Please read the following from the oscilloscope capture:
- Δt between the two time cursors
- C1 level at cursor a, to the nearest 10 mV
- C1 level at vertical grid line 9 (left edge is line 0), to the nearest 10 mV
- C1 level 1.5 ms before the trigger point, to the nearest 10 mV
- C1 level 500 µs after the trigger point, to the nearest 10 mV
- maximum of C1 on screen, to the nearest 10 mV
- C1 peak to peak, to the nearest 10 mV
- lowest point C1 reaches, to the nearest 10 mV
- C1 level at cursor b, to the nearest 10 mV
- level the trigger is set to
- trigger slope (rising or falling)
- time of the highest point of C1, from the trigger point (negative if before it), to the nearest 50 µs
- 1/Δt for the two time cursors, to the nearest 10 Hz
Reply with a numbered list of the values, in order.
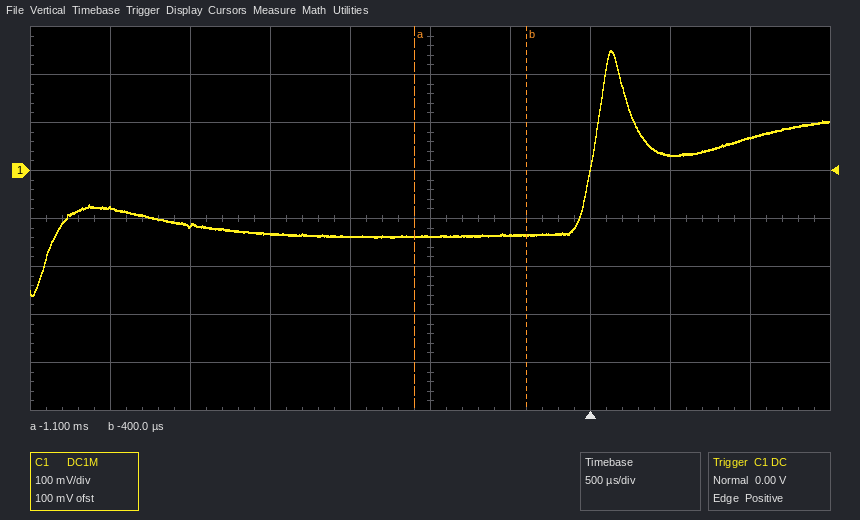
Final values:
1. 700 µs
2. -140 mV
3. 70 mV
4. -140 mV
5. 30 mV
6. 250 mV
7. 510 mV
8. -260 mV
9. -130 mV
10. 0.00 V
11. rising
12. +150 µs
13. 1.43 kHz
